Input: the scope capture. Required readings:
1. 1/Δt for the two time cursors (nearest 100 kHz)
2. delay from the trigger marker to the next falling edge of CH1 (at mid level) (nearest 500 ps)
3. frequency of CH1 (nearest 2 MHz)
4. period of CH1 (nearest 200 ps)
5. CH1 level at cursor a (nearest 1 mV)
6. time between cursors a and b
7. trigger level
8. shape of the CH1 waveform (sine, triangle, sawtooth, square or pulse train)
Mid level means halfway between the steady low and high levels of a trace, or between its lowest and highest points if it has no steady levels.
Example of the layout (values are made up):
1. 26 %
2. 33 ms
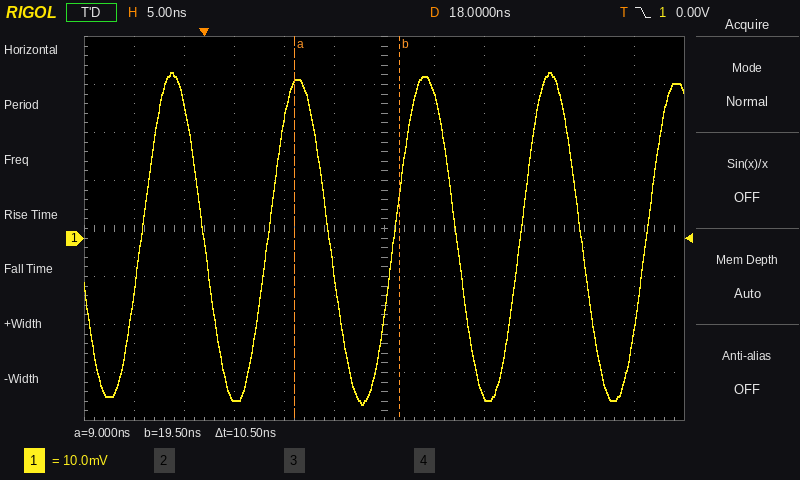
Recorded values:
1. 95.2 MHz
2. 12.5 ns
3. 80 MHz
4. 12.6 ns
5. 32 mV
6. 10.5 ns
7. 0.00 V
8. sine
